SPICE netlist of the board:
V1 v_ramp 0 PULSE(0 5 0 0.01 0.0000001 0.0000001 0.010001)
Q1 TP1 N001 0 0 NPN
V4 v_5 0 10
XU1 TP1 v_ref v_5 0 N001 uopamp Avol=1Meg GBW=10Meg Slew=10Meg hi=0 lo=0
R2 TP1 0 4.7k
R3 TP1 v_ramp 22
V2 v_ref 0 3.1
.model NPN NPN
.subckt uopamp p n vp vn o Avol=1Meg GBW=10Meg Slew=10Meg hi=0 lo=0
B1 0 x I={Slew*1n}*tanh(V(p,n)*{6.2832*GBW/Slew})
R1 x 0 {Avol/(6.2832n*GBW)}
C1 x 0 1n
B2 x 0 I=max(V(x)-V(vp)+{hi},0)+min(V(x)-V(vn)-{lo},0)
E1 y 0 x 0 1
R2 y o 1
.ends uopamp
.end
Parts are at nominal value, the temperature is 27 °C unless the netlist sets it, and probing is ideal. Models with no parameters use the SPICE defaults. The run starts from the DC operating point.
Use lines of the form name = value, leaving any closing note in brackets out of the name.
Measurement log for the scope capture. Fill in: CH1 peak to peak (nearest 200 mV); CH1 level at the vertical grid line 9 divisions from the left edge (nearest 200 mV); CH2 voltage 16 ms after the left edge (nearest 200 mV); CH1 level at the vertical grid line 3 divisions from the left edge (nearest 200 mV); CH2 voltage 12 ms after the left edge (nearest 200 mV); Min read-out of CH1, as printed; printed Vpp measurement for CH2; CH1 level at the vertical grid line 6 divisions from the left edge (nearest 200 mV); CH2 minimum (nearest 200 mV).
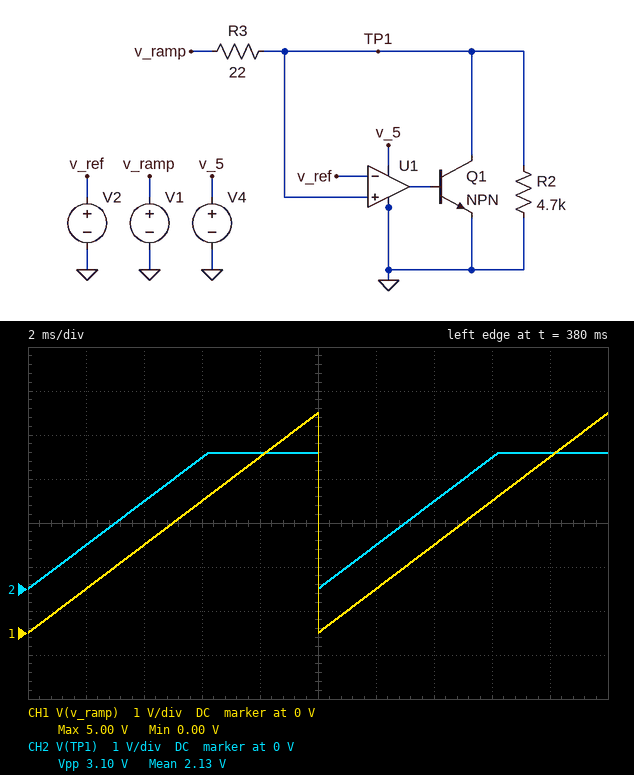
CH1 peak to peak = 5.0 V
CH1 level at the vertical grid line 9 divisions from the left edge = 4.0 V
CH2 voltage 16 ms after the left edge = 3.0 V
CH1 level at the vertical grid line 3 divisions from the left edge = 3.0 V
CH2 voltage 12 ms after the left edge = 1.0 V
Min read-out of CH1, as printed = 0.00 V
printed Vpp measurement for CH2 = 3.10 V
CH1 level at the vertical grid line 6 divisions from the left edge = 1.0 V
CH2 minimum = 0 V
